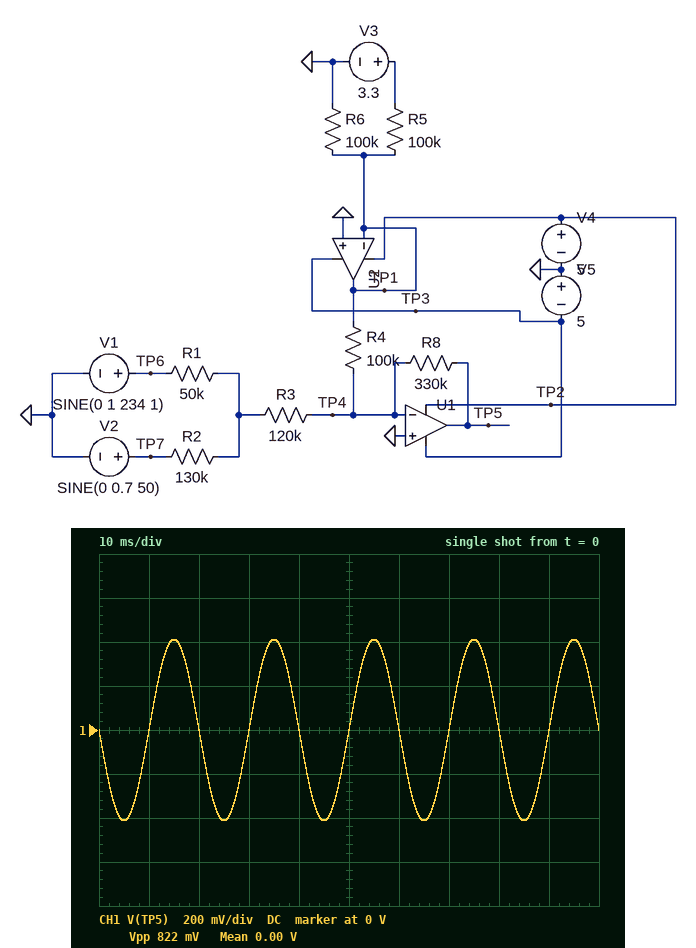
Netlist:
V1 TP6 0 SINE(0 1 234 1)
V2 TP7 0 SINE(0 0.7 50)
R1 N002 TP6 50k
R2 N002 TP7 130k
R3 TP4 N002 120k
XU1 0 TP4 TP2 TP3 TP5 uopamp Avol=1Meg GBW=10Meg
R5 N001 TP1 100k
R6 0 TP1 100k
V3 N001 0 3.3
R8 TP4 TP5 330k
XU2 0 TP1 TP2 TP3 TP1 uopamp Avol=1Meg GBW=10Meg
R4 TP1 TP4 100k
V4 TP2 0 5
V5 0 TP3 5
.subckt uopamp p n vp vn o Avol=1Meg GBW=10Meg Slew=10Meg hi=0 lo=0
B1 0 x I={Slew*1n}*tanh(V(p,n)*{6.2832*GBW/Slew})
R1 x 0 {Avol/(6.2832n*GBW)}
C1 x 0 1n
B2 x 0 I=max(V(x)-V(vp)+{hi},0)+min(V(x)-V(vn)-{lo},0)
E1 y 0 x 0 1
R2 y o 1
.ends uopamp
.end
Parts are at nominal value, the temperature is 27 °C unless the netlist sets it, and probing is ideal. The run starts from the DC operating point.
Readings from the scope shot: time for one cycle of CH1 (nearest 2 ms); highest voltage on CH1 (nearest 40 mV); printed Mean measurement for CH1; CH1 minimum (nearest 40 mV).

20 ms
400 mV
0.00 V
-400 mV
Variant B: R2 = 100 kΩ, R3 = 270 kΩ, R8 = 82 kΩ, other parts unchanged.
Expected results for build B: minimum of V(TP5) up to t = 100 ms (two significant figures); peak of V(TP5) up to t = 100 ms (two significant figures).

-63 mV
63 mV
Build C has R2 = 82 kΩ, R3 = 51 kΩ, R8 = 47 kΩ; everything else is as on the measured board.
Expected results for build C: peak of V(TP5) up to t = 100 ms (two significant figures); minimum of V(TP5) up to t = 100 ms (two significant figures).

150 mV
-150 mV
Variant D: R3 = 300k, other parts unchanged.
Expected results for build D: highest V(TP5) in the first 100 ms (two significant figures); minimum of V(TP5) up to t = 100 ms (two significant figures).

190 mV
-190 mV
